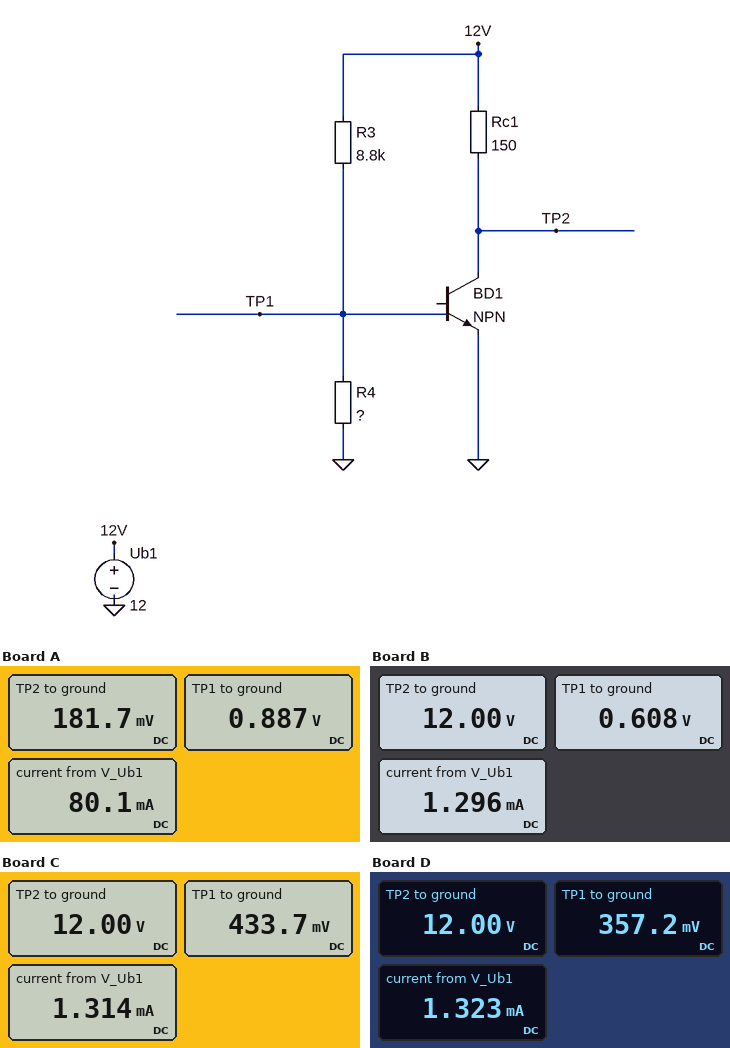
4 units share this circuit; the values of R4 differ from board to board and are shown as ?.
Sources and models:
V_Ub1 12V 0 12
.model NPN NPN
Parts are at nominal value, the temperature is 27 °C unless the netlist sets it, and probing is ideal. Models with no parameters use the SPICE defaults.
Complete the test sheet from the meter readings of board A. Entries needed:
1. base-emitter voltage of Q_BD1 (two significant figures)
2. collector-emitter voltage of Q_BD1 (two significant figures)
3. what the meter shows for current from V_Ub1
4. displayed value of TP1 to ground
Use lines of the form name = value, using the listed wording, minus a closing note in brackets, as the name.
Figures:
base-emitter voltage of Q_BD1 = 890 mV
collector-emitter voltage of Q_BD1 = 180 mV
what the meter shows for current from V_Ub1 = 80.1 mA
displayed value of TP1 to ground = 0.887 V
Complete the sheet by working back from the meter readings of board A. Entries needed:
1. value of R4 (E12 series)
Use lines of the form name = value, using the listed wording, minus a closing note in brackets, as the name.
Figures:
value of R4 = 2.2 kΩ
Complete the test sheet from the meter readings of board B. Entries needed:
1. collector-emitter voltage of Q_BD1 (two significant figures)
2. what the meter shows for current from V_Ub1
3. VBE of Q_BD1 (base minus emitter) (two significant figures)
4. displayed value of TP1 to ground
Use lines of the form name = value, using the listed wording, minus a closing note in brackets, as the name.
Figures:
collector-emitter voltage of Q_BD1 = 12 V
what the meter shows for current from V_Ub1 = 1.296 mA
VBE of Q_BD1 (base minus emitter) = 610 mV
displayed value of TP1 to ground = 0.608 V
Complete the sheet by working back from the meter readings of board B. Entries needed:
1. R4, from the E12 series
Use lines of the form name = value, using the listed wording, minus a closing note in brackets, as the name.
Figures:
R4, from the E12 series = 470 Ω
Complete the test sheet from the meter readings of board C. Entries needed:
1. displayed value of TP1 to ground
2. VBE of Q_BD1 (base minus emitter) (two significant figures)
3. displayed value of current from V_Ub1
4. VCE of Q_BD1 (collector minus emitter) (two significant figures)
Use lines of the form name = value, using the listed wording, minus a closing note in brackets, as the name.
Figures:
displayed value of TP1 to ground = 433.7 mV
VBE of Q_BD1 (base minus emitter) = 430 mV
displayed value of current from V_Ub1 = 1.314 mA
VCE of Q_BD1 (collector minus emitter) = 12 V
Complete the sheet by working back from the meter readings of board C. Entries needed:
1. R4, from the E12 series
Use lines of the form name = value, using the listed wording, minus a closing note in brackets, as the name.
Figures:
R4, from the E12 series = 330 Ω
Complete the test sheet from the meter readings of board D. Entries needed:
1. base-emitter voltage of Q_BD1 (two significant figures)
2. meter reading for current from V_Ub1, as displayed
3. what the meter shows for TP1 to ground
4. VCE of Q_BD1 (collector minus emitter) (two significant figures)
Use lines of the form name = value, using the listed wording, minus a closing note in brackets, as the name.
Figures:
base-emitter voltage of Q_BD1 = 360 mV
meter reading for current from V_Ub1, as displayed = 1.323 mA
what the meter shows for TP1 to ground = 357.2 mV
VCE of Q_BD1 (collector minus emitter) = 12 V
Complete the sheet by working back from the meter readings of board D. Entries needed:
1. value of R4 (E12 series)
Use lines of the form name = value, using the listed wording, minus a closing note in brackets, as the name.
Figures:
value of R4 = 270 Ω
